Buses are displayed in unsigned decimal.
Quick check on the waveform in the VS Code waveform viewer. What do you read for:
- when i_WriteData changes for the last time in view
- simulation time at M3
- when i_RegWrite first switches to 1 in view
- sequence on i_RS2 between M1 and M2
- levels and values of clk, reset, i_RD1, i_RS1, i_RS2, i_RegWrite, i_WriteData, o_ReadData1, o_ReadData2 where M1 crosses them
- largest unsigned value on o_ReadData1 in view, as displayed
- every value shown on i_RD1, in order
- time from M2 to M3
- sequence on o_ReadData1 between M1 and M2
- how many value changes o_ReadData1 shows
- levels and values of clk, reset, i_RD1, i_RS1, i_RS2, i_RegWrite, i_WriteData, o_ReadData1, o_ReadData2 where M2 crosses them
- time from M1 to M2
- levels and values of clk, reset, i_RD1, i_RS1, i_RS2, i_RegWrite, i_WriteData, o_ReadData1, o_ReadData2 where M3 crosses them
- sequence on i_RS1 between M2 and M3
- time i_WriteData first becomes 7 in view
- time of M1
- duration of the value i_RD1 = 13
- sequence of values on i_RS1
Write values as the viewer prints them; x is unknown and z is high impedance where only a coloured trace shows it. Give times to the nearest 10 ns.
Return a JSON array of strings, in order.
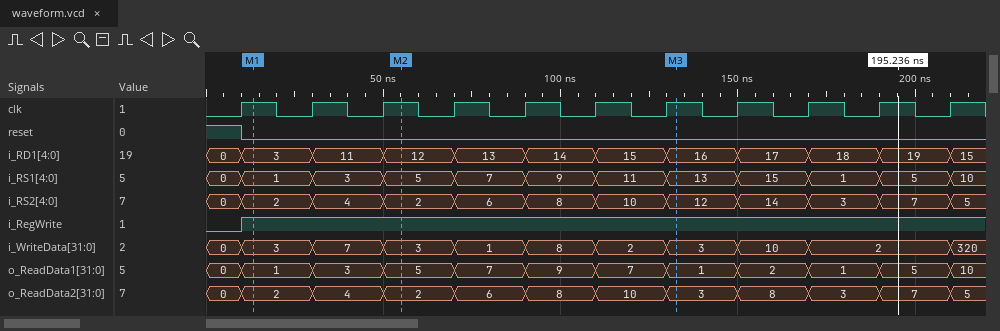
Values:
["210 ns", "130 ns", "10 ns", "2, 4, 2", "clk=1, reset=0, i_RD1=3, i_RS1=1, i_RS2=2, i_RegWrite=1, i_WriteData=3, o_ReadData1=1, o_ReadData2=2", "10", "0, 3, 11, 12, 13, 14, 15, 16, 17, 18, 19, 15", "80 ns", "1, 3, 5", "11", "clk=1, reset=0, i_RD1=12, i_RS1=5, i_RS2=2, i_RegWrite=1, i_WriteData=3, o_ReadData1=5, o_ReadData2=2", "40 ns", "clk=1, reset=0, i_RD1=16, i_RS1=13, i_RS2=12, i_RegWrite=1, i_WriteData=3, o_ReadData1=1, o_ReadData2=3", "5, 7, 9, 11, 13", "30 ns", "10 ns", "20 ns", "0, 1, 3, 5, 7, 9, 11, 13, 15, 1, 5, 10"]
